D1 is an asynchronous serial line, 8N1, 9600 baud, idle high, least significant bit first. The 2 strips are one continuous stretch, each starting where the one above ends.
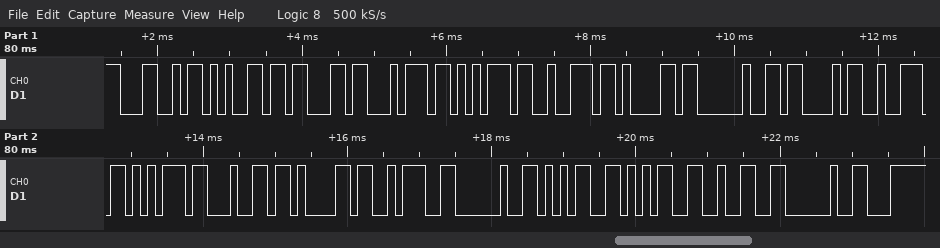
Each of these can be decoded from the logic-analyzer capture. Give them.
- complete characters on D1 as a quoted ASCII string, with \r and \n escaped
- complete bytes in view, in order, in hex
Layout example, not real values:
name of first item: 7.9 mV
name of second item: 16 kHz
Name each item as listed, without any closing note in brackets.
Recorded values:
complete characters on D1 as a quoted ASCII string, with \r and \n escaped: "Lectura Cruda: 552 "
complete bytes in view, in order, in hex: 4C 65 63 74 75 72 61 20 43 72 75 64 61 3A 20 35 35 32 20
